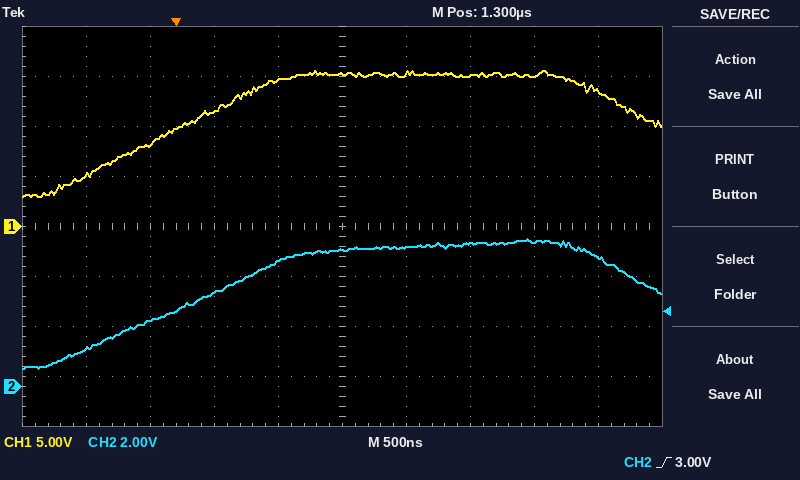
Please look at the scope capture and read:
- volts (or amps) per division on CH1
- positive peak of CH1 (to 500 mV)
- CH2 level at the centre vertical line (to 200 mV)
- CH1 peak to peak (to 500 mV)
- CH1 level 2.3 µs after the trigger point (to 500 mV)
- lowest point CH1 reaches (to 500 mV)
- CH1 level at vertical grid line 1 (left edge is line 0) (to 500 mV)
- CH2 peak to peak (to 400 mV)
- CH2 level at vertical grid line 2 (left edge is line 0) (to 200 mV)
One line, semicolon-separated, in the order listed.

5 V; 15.5 V; 5.4 V; 12.5 V; 15.0 V; 3.0 V; 5.0 V; 5.2 V; 2.6 V
